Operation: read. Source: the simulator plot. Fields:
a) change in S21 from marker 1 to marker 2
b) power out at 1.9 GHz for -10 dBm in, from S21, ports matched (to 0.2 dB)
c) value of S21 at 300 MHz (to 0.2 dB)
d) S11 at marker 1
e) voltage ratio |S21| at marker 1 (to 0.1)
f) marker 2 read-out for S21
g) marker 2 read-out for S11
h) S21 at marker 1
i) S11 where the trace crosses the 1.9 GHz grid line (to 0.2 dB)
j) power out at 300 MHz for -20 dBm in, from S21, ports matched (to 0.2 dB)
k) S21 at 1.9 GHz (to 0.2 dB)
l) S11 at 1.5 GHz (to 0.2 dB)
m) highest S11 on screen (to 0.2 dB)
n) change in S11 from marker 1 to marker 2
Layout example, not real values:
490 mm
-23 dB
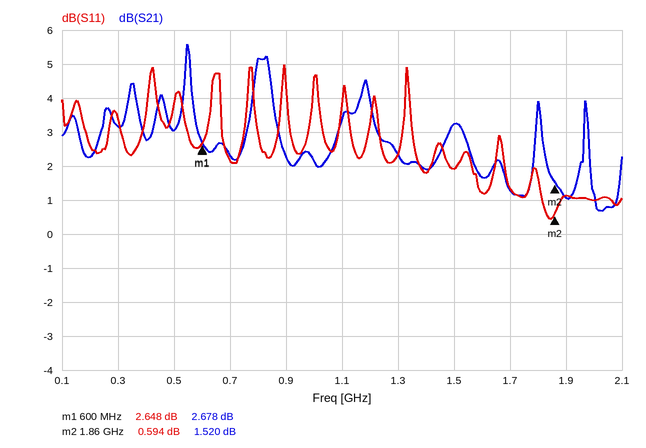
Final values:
-1.158 dB
-9.0 dBm
3.2 dB
2.648 dB
1.4
1.520 dB
0.594 dB
2.678 dB
1.2 dB
-16.8 dBm
1.0 dB
2.0 dB
5.0 dB
-2.054 dB
